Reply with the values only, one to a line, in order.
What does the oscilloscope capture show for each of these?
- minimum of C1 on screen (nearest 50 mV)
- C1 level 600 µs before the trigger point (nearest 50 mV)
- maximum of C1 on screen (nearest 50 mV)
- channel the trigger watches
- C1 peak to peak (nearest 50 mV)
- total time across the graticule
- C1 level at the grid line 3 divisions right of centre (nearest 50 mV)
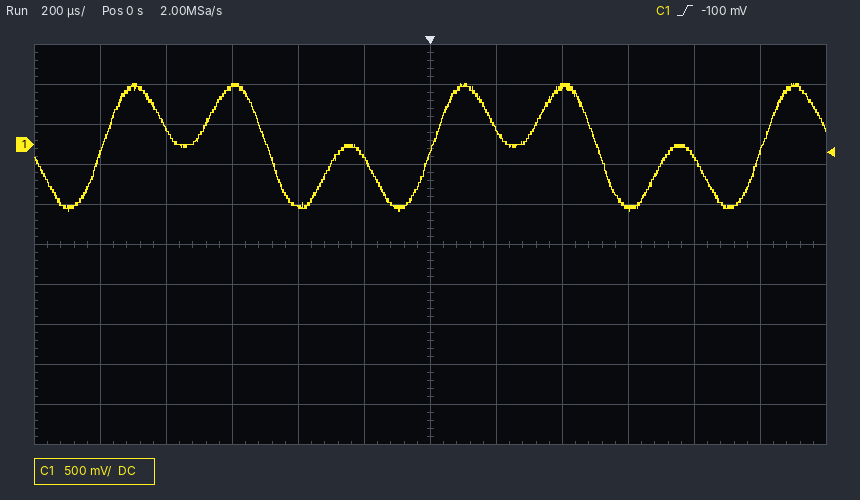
-850 mV
700 mV
750 mV
C1
1.60 V
2.4 ms
-800 mV
